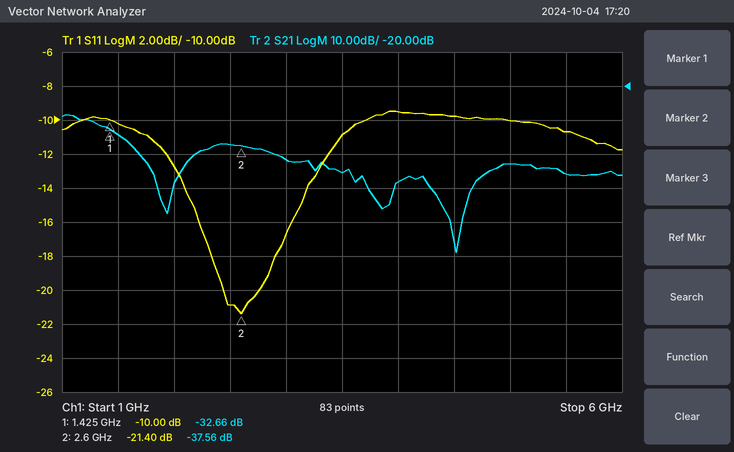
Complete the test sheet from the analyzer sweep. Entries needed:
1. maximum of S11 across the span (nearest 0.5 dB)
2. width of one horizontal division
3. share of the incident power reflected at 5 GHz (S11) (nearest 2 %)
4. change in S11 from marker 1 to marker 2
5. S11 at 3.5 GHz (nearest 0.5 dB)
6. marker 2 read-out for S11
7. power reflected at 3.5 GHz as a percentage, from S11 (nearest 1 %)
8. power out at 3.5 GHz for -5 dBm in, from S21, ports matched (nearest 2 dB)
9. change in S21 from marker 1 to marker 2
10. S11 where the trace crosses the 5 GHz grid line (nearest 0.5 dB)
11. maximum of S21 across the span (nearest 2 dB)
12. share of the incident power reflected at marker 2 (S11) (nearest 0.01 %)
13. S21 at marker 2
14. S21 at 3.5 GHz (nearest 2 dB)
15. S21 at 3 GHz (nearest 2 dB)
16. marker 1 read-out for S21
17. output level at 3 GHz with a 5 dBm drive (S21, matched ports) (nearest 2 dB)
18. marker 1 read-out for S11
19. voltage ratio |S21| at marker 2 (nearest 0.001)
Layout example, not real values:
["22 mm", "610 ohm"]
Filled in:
["-9.5 dB", "500 MHz", "10 %", "-11.40 dB", "-11.0 dB", "-21.40 dB", "8 %", "-50 dBm", "-4.90 dB", "-10.0 dB", "-28 dB", "0.72 %", "-37.56 dB", "-46 dB", "-42 dB", "-32.66 dB", "-36 dBm", "-10.00 dB", "0.013"]
